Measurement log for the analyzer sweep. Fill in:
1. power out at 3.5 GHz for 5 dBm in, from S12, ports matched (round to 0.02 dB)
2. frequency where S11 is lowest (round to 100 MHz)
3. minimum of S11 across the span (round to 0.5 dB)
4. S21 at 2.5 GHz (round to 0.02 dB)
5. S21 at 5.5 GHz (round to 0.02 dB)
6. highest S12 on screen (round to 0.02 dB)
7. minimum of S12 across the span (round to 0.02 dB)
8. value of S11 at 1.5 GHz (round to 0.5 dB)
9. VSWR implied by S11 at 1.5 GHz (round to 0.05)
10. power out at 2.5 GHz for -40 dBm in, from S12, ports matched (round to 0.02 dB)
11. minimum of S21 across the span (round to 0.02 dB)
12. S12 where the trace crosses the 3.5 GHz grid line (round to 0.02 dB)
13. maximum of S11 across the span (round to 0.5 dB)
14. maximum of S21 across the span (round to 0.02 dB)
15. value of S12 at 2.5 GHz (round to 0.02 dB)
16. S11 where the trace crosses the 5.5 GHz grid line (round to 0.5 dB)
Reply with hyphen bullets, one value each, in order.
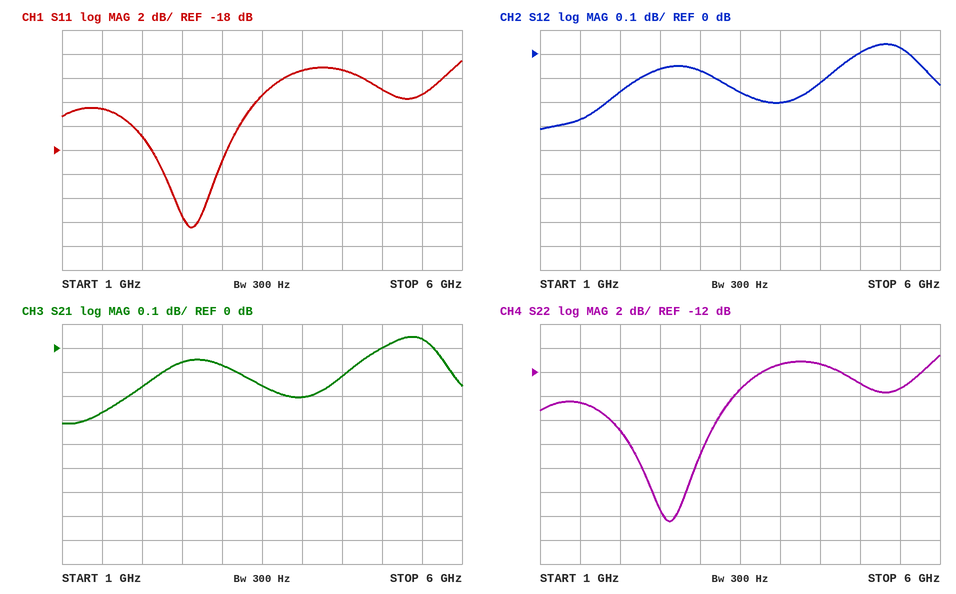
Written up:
- 4.84 dBm
- 2.6 GHz
- -24.5 dB
- -0.06 dB
- 0.04 dB
- 0.04 dB
- -0.32 dB
- -14.5 dB
- 1.45
- -40.06 dBm
- -0.32 dB
- -0.16 dB
- -10.5 dB
- 0.04 dB
- -0.06 dB
- -13.5 dB
